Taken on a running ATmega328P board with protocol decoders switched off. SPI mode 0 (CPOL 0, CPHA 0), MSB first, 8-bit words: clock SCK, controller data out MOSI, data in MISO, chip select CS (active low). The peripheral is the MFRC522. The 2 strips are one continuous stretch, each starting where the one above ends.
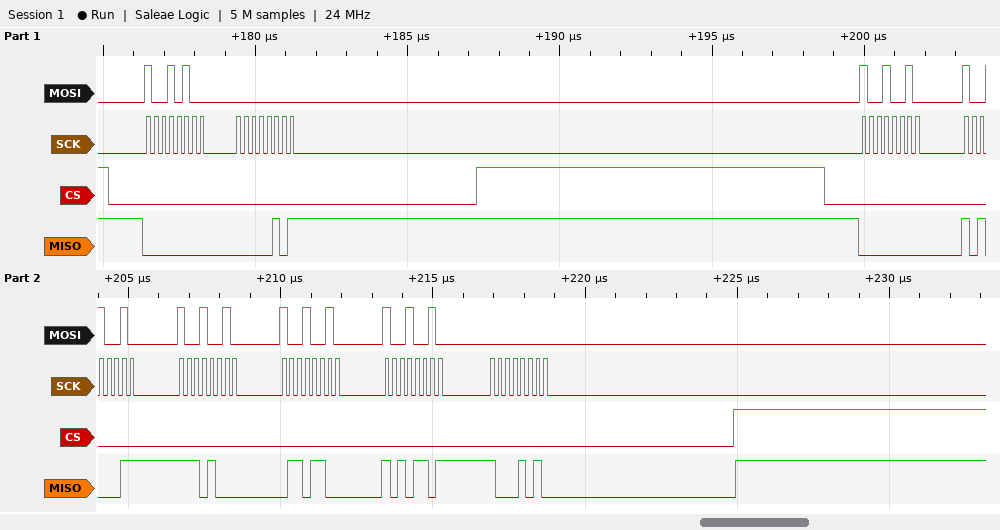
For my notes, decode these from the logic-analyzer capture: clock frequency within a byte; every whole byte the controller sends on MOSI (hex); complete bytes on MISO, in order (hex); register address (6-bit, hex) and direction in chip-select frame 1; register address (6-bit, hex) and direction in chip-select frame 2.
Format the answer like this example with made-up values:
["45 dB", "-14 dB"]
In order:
["4 MHz", "94 00 92 92 92 92 92 00", "00 05 00 A3 E8 6C AD 8A", "0x0A read", "0x09 read"]
